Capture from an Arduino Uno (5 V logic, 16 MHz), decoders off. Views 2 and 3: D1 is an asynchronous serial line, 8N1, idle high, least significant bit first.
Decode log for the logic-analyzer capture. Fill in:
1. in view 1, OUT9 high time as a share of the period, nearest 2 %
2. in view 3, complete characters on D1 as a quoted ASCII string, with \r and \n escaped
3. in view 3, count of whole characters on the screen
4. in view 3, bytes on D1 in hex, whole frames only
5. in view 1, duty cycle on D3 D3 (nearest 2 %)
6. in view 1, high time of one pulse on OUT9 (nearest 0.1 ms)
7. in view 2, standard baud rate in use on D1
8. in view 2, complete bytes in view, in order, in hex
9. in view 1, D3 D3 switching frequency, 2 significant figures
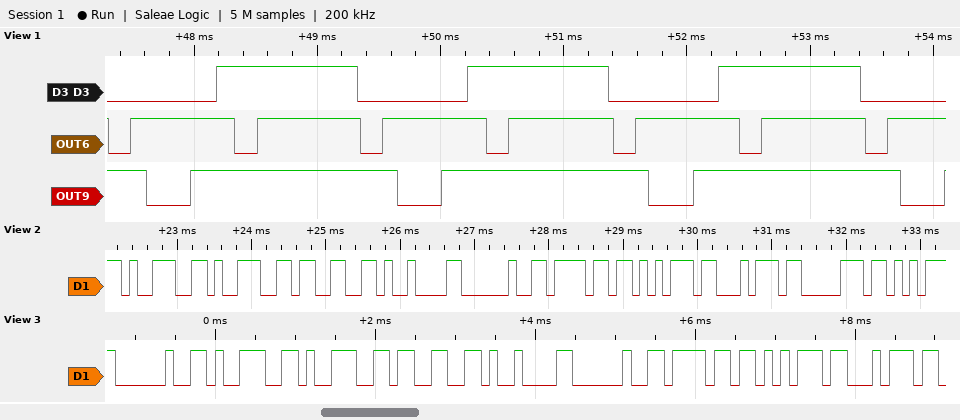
82 %
" 993\t out"
9
0x20 0x39 0x39 0x33 0x09 0x20 0x6F 0x75 0x74
56 %
1.7 ms
9600 baud
39 39 33 09 20 6F 75 74 70
490 Hz
